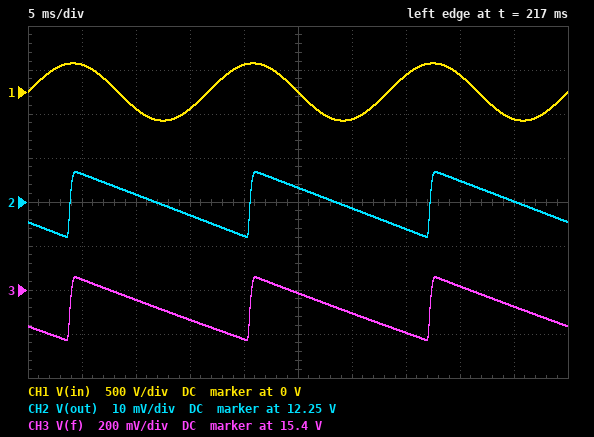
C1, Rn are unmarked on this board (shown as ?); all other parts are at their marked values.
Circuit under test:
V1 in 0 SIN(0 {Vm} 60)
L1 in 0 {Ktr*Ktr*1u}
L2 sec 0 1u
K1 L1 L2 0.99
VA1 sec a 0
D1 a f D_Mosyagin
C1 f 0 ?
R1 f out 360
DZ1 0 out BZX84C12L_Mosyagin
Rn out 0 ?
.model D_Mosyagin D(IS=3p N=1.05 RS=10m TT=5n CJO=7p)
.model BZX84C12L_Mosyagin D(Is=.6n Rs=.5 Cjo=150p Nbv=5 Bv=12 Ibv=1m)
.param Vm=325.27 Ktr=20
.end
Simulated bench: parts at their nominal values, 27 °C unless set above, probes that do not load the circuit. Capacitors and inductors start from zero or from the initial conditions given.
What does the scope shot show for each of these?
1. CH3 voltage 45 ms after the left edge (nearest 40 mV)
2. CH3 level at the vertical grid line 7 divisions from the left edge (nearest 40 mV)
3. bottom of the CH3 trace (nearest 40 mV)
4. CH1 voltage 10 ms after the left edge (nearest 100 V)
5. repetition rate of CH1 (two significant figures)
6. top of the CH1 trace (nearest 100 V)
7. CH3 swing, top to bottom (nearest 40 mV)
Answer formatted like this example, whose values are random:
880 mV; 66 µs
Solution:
15.32 V; 15.20 V; 15.16 V; -200 V; 60 Hz; 300 V; 280 mV
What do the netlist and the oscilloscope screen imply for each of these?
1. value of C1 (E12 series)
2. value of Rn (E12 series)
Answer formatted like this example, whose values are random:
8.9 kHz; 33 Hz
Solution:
470 µF; 6.8 kΩ
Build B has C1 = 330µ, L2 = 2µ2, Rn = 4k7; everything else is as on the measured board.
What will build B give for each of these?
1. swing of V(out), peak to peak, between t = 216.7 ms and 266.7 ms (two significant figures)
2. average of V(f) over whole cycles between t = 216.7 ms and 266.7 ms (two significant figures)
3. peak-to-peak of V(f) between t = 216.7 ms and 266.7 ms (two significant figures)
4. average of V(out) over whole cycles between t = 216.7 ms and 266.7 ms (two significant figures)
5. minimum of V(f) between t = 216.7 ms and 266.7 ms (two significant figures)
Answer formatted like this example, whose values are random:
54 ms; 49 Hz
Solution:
20 mV; 23 V; 1.3 V; 12 V; 22 V
